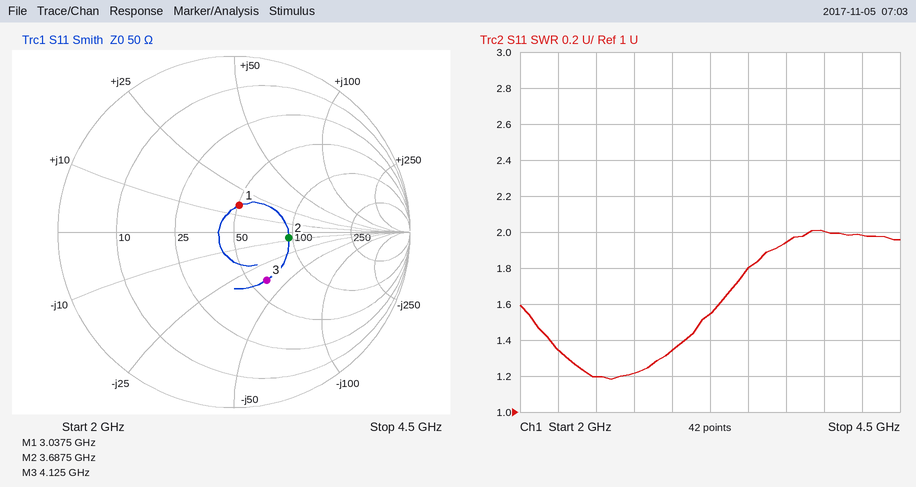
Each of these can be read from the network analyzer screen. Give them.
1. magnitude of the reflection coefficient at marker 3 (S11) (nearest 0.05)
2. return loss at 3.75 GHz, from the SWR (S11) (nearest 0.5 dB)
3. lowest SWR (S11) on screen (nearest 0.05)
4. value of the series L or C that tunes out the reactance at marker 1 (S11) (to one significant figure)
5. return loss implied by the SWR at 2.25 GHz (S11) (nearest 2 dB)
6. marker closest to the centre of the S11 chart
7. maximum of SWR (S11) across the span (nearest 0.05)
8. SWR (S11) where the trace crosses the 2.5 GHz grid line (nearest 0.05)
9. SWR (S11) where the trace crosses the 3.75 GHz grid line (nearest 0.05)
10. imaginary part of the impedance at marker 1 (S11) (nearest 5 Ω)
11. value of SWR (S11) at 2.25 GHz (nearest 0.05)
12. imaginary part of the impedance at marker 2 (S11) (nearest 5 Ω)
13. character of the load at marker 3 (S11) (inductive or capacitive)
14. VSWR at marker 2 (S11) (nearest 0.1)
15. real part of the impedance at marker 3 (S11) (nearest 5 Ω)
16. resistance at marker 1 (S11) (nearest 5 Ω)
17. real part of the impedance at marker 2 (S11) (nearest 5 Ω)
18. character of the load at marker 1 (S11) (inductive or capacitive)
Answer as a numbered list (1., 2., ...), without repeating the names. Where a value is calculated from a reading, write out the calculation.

1. 0.35
2. −20 log10((1.95 − 1)/(1.95 + 1)) ≈ 9.84 dB, so 10.0 dB to the nearest 0.5 dB
3. 1.20
4. C = 1/(2π × 3.0375 GHz × 15 Ω) ≈ 3 pF
5. −20 log10((1.35 − 1)/(1.35 + 1)) ≈ 16 dB
6. marker 1
7. 2.00
8. 1.20
9. 1.95
10. +15 Ω
11. 1.35
12. -5 Ω
13. capacitive
14. 1.9
15. 60 Ω
16. 50 Ω
17. 95 Ω
18. inductive
